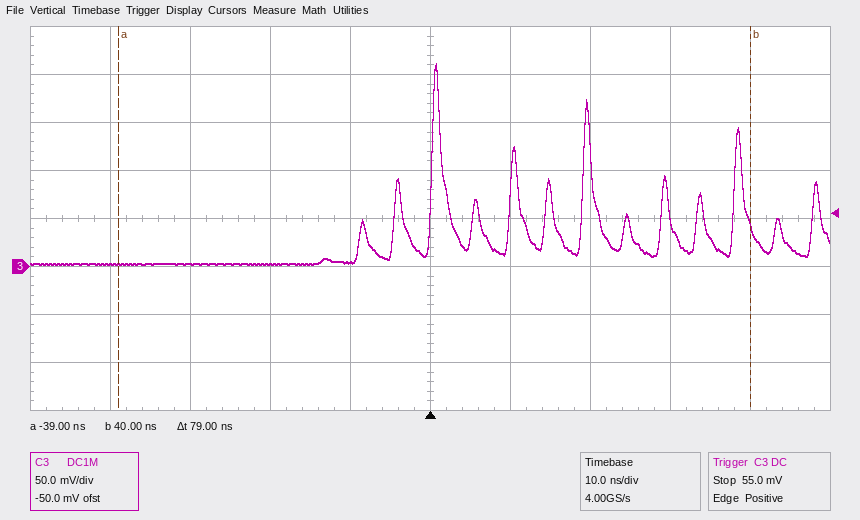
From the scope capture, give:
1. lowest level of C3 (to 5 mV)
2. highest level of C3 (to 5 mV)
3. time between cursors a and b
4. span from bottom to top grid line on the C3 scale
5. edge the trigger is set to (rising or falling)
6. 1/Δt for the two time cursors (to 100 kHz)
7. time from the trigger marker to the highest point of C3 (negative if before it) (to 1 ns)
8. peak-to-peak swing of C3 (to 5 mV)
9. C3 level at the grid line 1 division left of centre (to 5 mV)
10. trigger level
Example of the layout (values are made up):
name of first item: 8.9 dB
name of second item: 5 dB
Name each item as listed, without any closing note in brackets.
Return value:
lowest level of C3: 0 mV
highest level of C3: 210 mV
time between cursors a and b: 79 ns
span from bottom to top grid line on the C3 scale: 400 mV
edge the trigger is set to: rising
1/Δt for the two time cursors: 12.7 MHz
time from the trigger marker to the highest point of C3 (negative if before it): +1 ns
peak-to-peak swing of C3: 210 mV
C3 level at the grid line 1 division left of centre: 5 mV
trigger level: 55.0 mV
